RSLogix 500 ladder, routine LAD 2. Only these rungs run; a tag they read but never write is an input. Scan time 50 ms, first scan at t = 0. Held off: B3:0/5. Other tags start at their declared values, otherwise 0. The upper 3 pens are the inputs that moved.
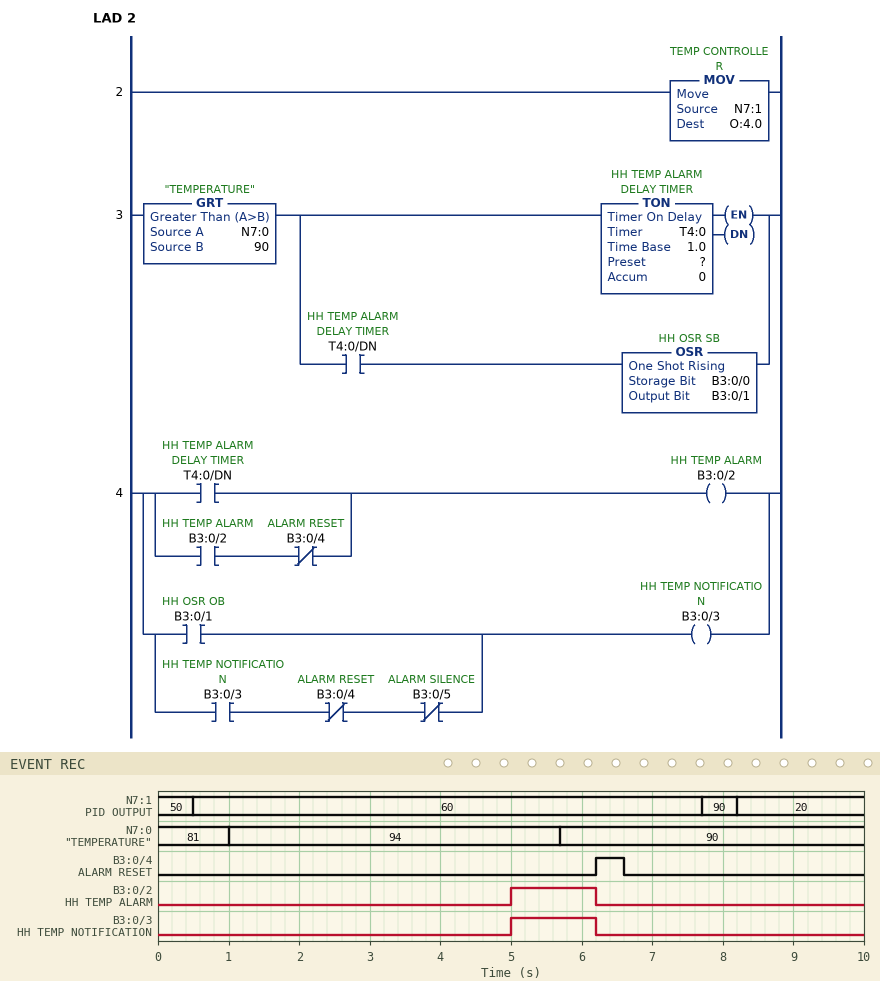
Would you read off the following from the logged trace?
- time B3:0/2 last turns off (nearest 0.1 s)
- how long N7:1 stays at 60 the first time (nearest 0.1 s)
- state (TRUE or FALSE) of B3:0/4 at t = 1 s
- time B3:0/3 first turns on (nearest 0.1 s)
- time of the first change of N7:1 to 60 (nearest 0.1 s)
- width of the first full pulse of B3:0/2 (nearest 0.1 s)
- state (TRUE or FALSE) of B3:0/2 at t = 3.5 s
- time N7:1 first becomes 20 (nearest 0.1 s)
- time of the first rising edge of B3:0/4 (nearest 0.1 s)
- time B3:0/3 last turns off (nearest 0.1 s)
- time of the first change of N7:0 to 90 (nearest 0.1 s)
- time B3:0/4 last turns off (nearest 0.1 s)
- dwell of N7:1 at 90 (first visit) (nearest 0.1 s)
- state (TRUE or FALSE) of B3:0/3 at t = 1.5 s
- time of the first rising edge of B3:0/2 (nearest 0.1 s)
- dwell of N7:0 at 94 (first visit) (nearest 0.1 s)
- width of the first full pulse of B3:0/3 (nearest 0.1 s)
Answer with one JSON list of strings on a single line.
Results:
["6.2 s", "7.2 s", "FALSE", "5.0 s", "0.5 s", "1.2 s", "FALSE", "8.2 s", "6.2 s", "6.2 s", "5.7 s", "6.6 s", "0.5 s", "FALSE", "5.0 s", "4.7 s", "1.2 s"]
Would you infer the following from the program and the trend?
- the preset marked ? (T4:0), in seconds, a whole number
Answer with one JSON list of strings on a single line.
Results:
["4 s"]
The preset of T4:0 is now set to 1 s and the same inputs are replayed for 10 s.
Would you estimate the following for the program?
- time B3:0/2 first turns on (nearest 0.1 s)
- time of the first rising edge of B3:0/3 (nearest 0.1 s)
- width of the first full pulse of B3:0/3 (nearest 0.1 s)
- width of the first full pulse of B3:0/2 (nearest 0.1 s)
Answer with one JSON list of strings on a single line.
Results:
["2.0 s", "2.0 s", "4.2 s", "4.2 s"]
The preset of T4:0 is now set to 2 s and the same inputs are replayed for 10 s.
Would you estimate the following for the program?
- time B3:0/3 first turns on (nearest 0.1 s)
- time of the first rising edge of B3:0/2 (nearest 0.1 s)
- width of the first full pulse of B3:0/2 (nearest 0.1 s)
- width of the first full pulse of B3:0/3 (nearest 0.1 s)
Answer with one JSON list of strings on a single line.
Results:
["3.0 s", "3.0 s", "3.2 s", "3.2 s"]
